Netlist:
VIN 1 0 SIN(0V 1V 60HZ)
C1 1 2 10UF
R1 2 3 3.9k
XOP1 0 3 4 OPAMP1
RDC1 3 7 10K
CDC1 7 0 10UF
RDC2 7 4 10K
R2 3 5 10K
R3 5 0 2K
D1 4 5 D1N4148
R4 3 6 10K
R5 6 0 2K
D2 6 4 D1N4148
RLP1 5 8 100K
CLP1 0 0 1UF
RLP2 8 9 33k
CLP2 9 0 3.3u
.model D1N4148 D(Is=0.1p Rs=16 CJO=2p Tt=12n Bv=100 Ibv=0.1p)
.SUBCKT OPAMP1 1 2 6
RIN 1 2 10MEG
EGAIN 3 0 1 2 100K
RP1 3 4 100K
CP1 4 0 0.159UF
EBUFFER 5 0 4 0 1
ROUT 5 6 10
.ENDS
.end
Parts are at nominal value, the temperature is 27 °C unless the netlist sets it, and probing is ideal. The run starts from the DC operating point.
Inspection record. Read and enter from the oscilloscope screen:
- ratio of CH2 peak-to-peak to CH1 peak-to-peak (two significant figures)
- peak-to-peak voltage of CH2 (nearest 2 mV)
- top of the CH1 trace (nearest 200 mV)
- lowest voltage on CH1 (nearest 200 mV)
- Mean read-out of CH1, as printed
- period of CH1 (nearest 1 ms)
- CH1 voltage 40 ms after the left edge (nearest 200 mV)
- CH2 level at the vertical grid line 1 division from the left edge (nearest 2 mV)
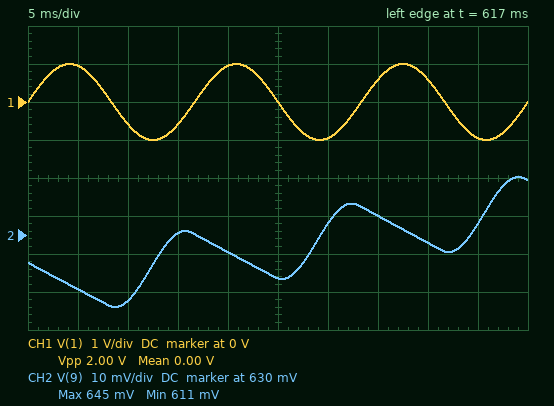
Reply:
0.017
34 mV
1.0 V
-1.0 V
0.00 V
17 ms
600 mV
616 mV
